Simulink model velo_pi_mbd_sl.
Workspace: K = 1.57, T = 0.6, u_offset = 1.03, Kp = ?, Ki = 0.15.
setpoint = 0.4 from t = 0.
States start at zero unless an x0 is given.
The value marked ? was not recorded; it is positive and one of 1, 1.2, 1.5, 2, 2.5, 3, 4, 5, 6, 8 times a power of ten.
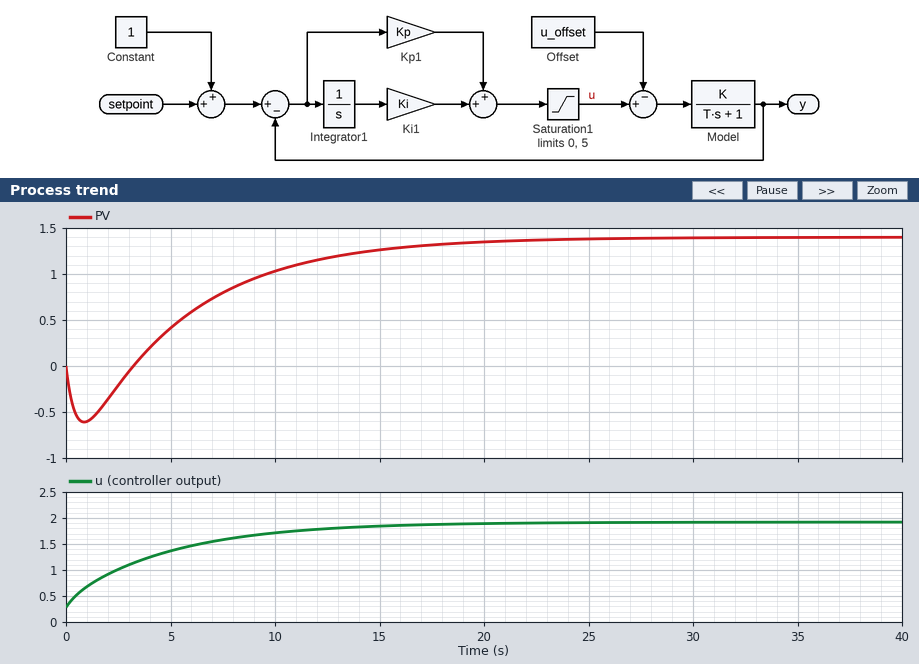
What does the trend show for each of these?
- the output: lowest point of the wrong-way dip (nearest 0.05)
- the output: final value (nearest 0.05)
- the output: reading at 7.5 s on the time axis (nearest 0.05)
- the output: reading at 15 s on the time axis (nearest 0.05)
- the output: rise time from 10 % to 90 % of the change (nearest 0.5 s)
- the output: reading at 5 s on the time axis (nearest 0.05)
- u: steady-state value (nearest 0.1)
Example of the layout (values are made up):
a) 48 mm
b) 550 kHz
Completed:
a) -0.60
b) 1.40
c) 0.80
d) 1.25
e) 11.0 s
f) 0.40
g) 1.9
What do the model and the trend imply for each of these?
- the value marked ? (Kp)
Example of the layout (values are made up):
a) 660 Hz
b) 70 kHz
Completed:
a) 0.2
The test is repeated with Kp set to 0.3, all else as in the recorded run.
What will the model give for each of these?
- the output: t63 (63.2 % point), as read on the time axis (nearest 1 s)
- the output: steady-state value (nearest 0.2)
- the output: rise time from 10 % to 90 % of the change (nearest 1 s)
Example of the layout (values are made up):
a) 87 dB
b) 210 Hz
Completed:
a) 9 s
b) 1.4
c) 13 s
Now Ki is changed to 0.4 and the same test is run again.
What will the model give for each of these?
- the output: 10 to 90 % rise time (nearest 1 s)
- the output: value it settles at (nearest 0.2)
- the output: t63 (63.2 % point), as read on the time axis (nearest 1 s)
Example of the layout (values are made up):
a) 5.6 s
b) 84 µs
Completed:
a) 3 s
b) 1.4
c) 3 s
